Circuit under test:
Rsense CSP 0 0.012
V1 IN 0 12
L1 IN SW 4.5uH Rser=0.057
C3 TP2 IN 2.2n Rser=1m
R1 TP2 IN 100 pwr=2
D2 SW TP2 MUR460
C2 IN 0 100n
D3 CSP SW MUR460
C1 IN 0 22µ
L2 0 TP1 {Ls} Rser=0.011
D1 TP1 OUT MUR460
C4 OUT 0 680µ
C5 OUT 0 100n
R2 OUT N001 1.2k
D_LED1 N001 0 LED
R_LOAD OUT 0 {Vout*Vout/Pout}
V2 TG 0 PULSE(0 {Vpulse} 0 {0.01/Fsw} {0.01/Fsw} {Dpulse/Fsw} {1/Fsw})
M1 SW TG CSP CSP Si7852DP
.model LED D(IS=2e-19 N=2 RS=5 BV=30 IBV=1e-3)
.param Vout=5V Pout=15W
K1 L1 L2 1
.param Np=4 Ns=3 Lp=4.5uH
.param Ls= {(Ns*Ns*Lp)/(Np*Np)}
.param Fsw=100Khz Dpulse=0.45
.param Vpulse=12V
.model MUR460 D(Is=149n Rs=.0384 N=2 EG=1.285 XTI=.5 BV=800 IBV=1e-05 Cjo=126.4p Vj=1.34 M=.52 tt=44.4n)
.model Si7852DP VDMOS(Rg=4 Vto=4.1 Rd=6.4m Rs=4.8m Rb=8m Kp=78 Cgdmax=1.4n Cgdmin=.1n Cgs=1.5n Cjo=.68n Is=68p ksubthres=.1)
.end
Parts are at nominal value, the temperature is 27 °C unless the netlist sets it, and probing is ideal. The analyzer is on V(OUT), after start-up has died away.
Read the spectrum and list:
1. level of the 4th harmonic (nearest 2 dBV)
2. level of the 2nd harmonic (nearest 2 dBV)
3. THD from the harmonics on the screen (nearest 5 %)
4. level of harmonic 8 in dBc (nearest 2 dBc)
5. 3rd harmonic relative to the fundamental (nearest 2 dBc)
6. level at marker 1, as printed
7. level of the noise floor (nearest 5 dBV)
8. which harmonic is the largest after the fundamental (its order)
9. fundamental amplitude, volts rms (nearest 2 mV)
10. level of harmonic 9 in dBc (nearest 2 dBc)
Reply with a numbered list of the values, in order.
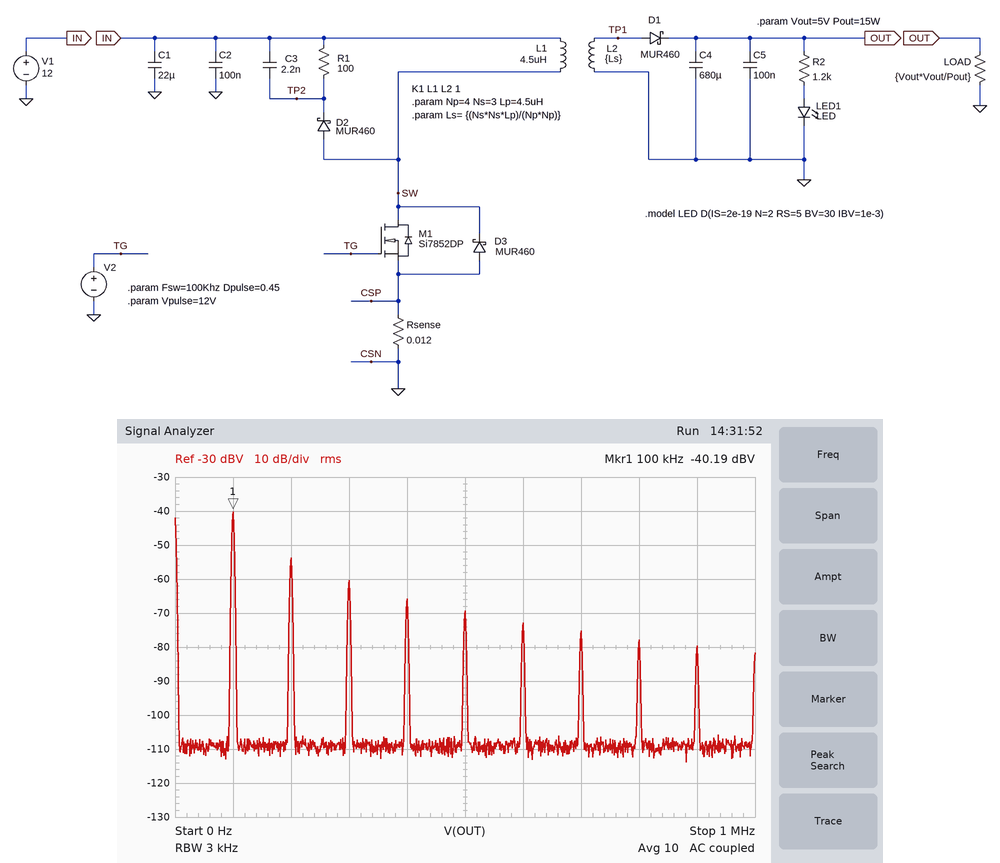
1. -66 dBV
2. -54 dBV
3. 25 %
4. -38 dBc
5. -20 dBc
6. -40.19 dBV
7. -110 dBV
8. 2
9. 10 mV
10. -40 dBc
